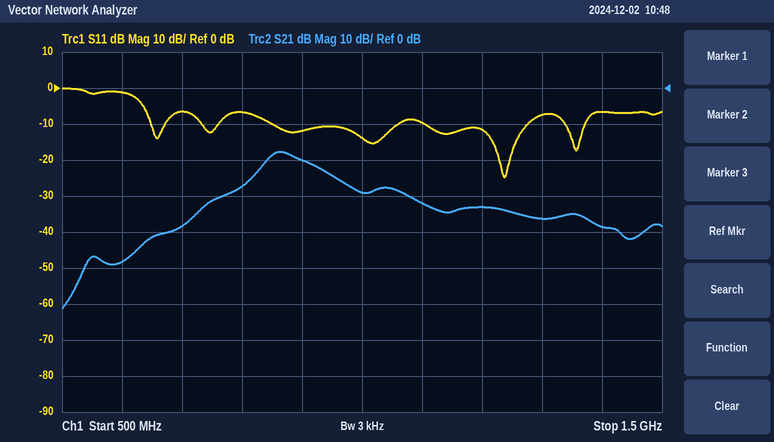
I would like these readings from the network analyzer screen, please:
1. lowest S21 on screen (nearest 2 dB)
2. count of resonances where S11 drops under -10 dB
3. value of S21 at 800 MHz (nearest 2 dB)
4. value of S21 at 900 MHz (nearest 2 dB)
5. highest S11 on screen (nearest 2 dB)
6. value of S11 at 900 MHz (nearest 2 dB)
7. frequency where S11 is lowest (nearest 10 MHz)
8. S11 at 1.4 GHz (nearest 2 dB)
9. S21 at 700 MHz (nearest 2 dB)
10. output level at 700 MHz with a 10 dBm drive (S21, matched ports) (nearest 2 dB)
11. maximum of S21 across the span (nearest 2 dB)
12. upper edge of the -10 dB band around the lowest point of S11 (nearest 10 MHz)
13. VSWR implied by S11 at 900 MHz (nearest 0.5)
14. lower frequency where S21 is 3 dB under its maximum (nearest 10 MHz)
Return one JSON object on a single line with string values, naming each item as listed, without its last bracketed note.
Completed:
{"lowest S21 on screen": "-62 dB", "count of resonances where S11 drops under -10 dB": "5", "value of S21 at 800 MHz": "-28 dB", "value of S21 at 900 MHz": "-20 dB", "highest S11 on screen": "0 dB", "value of S11 at 900 MHz": "-12 dB", "frequency where S11 is lowest": "1.24 GHz", "S11 at 1.4 GHz": "-6 dB", "S21 at 700 MHz": "-38 dB", "output level at 700 MHz with a 10 dBm drive (S21, matched ports)": "-28 dBm", "maximum of S21 across the span": "-18 dB", "upper edge of the -10 dB band around the lowest point of S11": "1.28 GHz", "VSWR implied by S11 at 900 MHz": "1.5", "lower frequency where S21 is 3 dB under its maximum": "840 MHz"}
